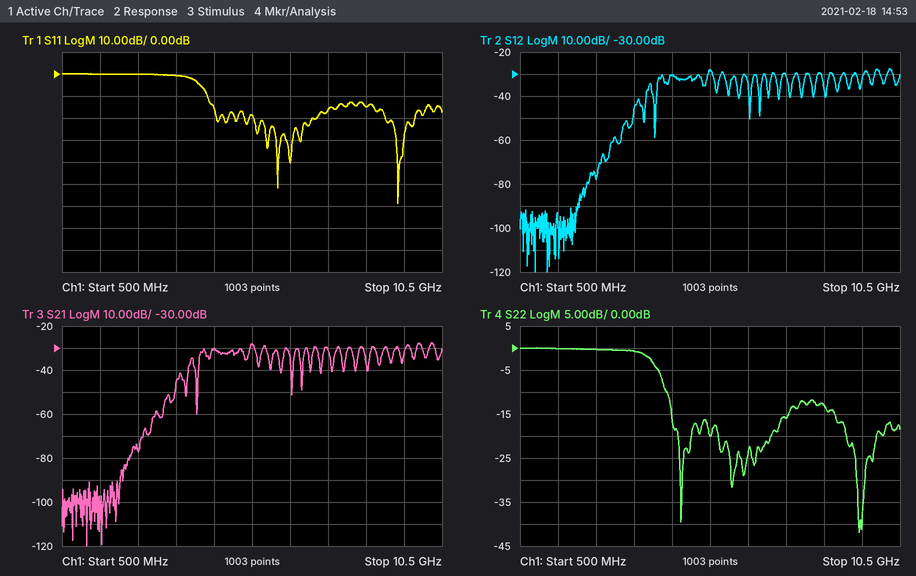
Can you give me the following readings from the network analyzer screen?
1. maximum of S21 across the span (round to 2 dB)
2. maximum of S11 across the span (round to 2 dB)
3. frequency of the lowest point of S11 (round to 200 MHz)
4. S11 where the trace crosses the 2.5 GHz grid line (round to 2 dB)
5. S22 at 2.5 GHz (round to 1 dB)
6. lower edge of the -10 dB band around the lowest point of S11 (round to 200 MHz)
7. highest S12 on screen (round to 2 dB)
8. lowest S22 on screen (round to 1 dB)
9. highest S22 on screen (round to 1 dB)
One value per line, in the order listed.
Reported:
-28 dB
0 dB
9.4 GHz
0 dB
0 dB
4.4 GHz
-28 dB
-42 dB
0 dB
